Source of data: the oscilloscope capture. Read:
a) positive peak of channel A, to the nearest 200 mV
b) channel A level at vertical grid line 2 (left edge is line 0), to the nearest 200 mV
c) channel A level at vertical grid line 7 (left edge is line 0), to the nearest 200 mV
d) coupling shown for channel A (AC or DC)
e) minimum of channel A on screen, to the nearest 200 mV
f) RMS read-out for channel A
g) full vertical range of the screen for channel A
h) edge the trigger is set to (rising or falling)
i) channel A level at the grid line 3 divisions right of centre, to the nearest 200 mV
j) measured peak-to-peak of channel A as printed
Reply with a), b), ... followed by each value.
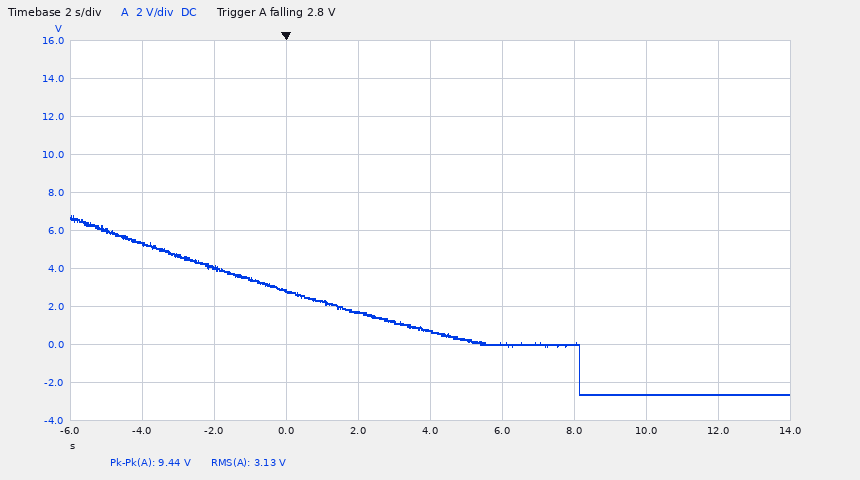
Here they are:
a) 6.8 V
b) 4.0 V
c) 0.0 V
d) DC
e) -2.6 V
f) 3.13 V
g) 20 V
h) falling
i) -2.6 V
j) 9.44 V
